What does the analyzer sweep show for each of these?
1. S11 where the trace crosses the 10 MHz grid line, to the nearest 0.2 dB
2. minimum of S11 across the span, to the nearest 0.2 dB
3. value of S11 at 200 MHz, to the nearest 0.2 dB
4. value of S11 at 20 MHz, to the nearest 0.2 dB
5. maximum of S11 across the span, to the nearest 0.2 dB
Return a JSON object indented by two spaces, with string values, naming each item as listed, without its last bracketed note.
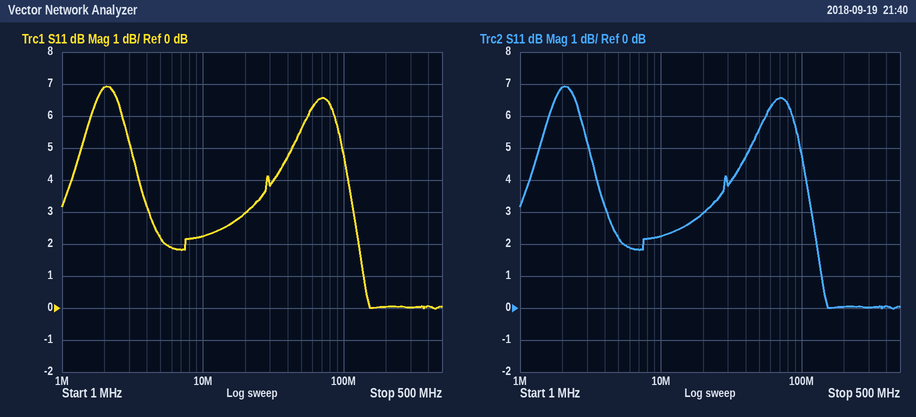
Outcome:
{
  "S11 where the trace crosses the 10 MHz grid line, to the nearest 0.2 dB": "2.2 dB",
  "minimum of S11 across the span, to the nearest 0.2 dB": "0.0 dB",
  "value of S11 at 200 MHz, to the nearest 0.2 dB": "0.0 dB",
  "value of S11 at 20 MHz, to the nearest 0.2 dB": "3.0 dB",
  "maximum of S11 across the span, to the nearest 0.2 dB": "7.0 dB"
}
